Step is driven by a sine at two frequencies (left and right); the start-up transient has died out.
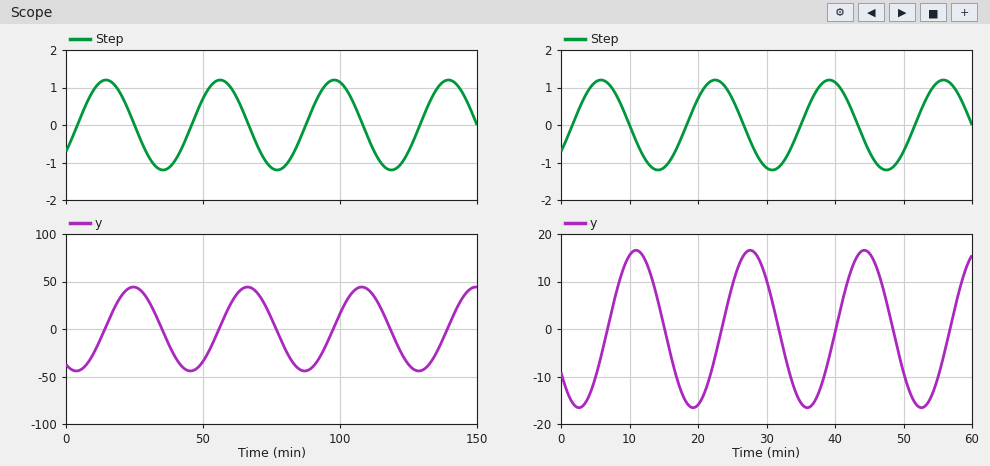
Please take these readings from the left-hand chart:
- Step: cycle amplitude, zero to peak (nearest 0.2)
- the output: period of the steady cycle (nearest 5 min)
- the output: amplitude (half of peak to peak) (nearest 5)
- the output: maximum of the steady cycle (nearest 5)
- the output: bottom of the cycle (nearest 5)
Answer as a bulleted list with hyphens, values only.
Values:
- 1.2
- 40 min
- 45
- 45
- -45
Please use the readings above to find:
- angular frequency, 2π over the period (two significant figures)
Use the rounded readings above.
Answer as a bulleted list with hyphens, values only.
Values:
- 0.16 rad/min
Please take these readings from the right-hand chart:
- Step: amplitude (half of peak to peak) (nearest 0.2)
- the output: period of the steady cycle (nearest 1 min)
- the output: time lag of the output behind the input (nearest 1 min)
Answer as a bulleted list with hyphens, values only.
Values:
- 1.2
- 17 min
- 5 min
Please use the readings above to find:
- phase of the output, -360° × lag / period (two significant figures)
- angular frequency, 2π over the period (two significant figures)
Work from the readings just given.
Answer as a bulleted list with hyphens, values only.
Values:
- -110°
- 0.37 rad/min
